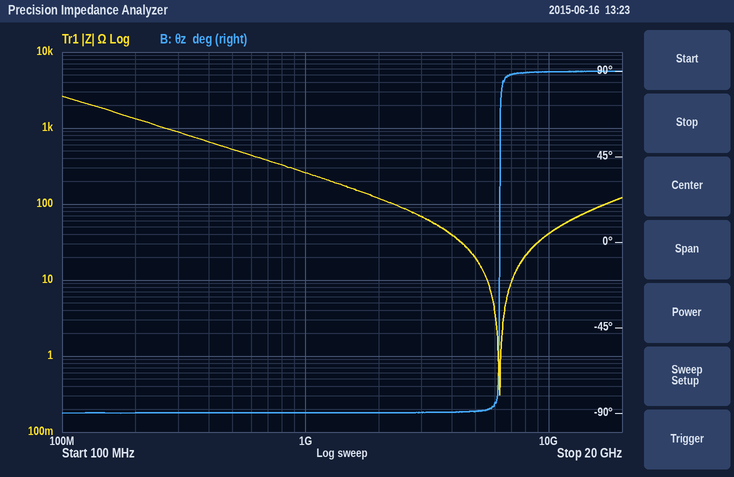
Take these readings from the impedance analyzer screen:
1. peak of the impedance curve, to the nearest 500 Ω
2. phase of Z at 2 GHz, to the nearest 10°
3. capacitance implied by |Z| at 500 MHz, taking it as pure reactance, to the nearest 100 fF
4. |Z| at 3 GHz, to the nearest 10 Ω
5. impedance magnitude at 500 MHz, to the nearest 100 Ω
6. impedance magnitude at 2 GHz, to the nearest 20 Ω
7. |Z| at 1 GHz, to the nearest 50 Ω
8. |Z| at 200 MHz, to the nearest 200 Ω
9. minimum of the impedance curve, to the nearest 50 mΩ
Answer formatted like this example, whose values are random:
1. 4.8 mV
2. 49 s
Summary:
1. 2.5 kΩ
2. -90°
3. 600 fF
4. 70 Ω
5. 500 Ω
6. 120 Ω
7. 250 Ω
8. 1.4 kΩ
9. 300 mΩ
